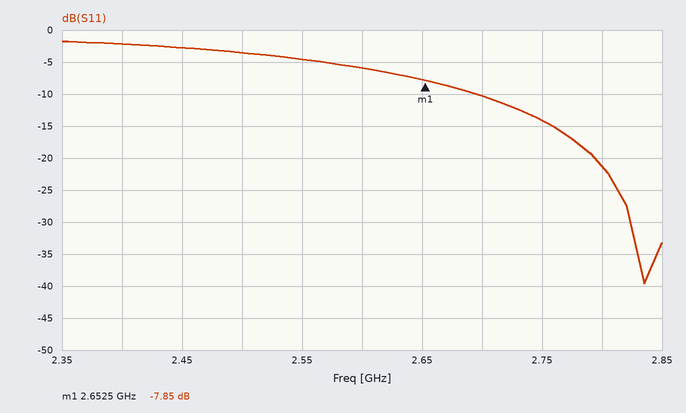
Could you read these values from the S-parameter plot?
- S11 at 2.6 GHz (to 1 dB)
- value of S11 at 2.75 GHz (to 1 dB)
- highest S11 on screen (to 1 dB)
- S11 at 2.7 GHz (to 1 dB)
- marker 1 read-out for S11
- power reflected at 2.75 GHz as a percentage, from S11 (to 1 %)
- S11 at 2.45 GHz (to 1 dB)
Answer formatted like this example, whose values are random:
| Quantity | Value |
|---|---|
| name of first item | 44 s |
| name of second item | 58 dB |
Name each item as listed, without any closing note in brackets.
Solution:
| Quantity | Value |
|---|---|
| S11 at 2.6 GHz | -6 dB |
| value of S11 at 2.75 GHz | -14 dB |
| highest S11 on screen | -2 dB |
| S11 at 2.7 GHz | -10 dB |
| marker 1 read-out for S11 | -7.85 dB |
| power reflected at 2.75 GHz as a percentage, from S11 | 4 % |
| S11 at 2.45 GHz | -3 dB |
